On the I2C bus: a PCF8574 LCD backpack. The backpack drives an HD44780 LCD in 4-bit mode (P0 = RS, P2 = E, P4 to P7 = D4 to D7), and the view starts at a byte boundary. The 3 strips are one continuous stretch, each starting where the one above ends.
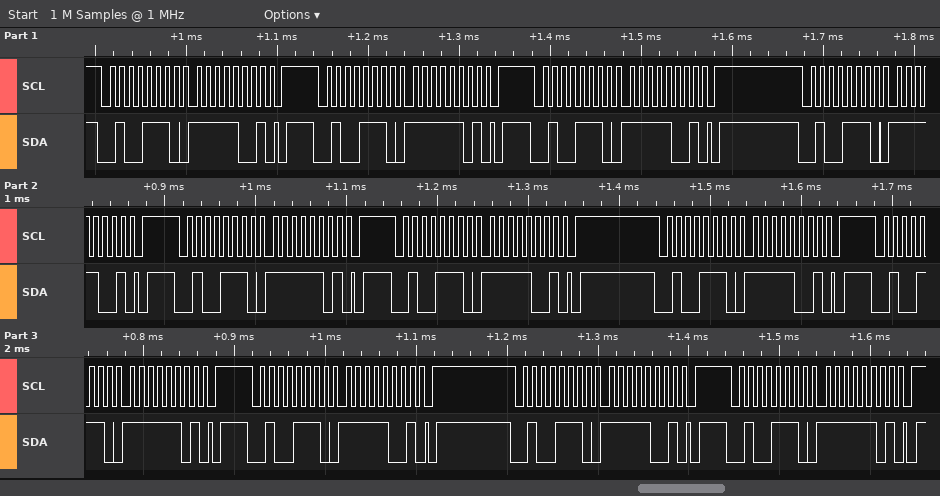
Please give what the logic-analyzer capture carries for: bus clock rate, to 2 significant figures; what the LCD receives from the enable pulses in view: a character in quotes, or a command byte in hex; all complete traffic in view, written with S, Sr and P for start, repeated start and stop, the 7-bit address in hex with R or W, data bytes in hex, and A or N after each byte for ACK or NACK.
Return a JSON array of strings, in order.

["100 kHz", "data 0xFF", "S 27W A F9 A P S 27W A FD A P S 27W A F9 A P S 27W A F9 A P S 27W A FD A P S 27W A F9 A P S 27W A F9 A P S 27W A FD A P S 27W A F9 A P S 27W A F9 A P S 27W A FD A P"]
